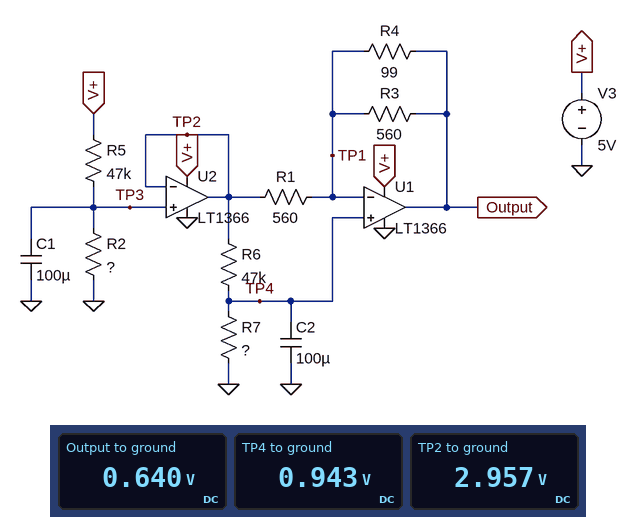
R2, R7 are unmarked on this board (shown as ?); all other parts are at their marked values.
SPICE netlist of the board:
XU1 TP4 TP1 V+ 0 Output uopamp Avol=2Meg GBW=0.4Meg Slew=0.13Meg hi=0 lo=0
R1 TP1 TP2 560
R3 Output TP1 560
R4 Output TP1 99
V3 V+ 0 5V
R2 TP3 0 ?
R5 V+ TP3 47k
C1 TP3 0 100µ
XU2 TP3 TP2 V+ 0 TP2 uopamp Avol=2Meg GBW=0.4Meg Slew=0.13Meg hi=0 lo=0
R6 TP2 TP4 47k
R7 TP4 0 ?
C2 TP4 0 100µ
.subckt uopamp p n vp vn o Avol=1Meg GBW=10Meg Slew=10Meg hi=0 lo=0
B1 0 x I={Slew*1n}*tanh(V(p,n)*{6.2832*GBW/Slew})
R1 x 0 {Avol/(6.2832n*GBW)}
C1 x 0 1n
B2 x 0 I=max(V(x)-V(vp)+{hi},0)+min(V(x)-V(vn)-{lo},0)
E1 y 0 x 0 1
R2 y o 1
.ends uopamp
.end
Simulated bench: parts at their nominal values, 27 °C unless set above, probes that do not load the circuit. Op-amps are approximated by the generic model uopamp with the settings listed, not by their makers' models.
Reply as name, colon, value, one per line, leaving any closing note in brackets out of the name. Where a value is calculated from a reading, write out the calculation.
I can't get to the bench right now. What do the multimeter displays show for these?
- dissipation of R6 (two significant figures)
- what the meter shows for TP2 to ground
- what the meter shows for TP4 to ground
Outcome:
dissipation of R6: (2.957 V - 943 mV)^2 / 47 kΩ = 86 µW
what the meter shows for TP2 to ground: 2.957 V
what the meter shows for TP4 to ground: 0.943 V
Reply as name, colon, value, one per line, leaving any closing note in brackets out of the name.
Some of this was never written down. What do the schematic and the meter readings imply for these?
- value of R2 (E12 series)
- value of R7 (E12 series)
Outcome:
value of R2: 68 kΩ
value of R7: 22 kΩ
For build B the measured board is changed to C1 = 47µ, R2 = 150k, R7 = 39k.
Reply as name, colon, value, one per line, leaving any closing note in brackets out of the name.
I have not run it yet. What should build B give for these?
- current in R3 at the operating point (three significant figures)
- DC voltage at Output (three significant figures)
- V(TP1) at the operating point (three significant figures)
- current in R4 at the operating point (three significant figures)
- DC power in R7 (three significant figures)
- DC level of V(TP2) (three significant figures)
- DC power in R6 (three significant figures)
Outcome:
current in R3 at the operating point: 558 µA
DC voltage at Output: 1.41 V
V(TP1) at the operating point: 1.73 V
current in R4 at the operating point: 3.16 mA
DC power in R7: 76.4 µW
DC level of V(TP2): 3.81 V
DC power in R6: 92.1 µW
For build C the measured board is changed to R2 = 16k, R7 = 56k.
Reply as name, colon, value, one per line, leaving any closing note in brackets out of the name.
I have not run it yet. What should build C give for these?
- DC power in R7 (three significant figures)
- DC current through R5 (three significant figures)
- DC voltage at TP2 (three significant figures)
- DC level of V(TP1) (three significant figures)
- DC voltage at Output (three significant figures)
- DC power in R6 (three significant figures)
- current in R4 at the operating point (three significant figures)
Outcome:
DC power in R7: 8.51 µW
DC current through R5: 79.4 µA
DC voltage at TP2: 1.27 V
DC level of V(TP1): 690 mV
DC voltage at Output: 603 mV
DC power in R6: 7.14 µW
current in R4 at the operating point: 879 µA
